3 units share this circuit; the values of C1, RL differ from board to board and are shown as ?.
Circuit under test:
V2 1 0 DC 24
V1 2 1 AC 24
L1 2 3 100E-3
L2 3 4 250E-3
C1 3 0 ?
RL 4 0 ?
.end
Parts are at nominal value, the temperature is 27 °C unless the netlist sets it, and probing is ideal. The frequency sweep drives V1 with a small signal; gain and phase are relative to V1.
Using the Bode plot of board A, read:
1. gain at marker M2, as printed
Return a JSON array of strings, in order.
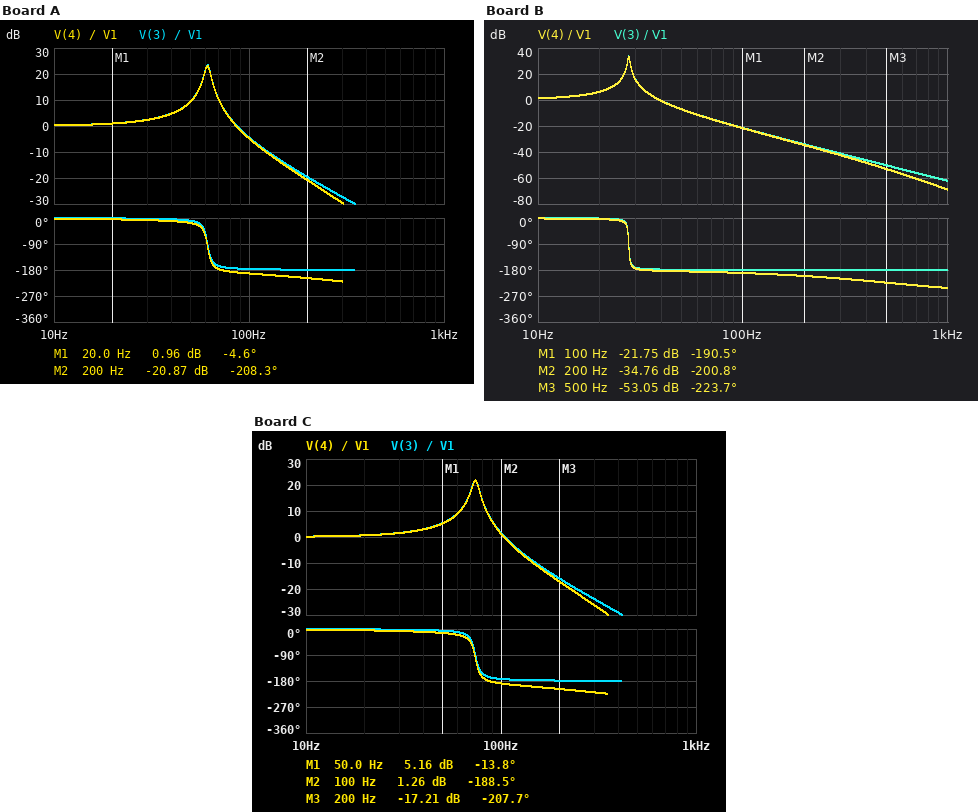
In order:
["-20.87 dB"]
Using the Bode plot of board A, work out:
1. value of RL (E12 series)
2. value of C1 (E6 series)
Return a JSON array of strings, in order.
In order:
["560 Ω", "68 µF"]
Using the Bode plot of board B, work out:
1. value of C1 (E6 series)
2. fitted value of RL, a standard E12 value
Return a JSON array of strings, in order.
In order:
["330 µF", "820 Ω"]
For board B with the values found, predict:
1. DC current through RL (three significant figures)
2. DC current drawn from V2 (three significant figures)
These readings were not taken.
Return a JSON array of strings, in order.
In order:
["29.3 mA", "29.3 mA"]
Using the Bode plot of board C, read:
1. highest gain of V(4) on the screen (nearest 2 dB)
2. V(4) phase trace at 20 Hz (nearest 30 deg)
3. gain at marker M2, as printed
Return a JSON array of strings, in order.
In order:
["22 dB", "0 deg", "1.26 dB"]
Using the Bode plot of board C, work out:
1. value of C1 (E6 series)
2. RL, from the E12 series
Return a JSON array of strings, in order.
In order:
["47 µF", "560 Ω"]
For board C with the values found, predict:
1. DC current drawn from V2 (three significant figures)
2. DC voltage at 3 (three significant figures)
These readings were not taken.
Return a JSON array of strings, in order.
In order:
["42.9 mA", "24.0 V"]
